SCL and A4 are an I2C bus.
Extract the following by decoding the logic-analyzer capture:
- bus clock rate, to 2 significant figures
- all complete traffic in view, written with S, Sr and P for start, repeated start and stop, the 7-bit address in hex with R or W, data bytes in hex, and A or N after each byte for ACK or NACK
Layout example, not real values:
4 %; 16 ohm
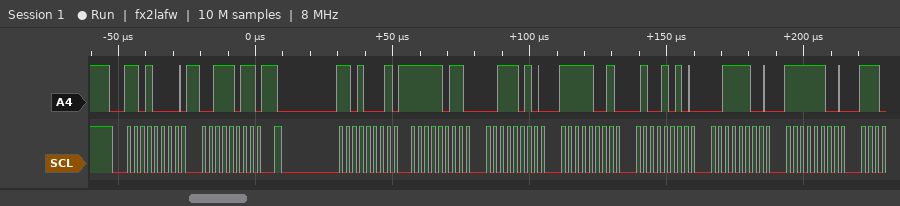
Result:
400 kHz; S 68W A 3B A Sr 68R A FB A 3A A F9 A 4A A 3C A FC A
